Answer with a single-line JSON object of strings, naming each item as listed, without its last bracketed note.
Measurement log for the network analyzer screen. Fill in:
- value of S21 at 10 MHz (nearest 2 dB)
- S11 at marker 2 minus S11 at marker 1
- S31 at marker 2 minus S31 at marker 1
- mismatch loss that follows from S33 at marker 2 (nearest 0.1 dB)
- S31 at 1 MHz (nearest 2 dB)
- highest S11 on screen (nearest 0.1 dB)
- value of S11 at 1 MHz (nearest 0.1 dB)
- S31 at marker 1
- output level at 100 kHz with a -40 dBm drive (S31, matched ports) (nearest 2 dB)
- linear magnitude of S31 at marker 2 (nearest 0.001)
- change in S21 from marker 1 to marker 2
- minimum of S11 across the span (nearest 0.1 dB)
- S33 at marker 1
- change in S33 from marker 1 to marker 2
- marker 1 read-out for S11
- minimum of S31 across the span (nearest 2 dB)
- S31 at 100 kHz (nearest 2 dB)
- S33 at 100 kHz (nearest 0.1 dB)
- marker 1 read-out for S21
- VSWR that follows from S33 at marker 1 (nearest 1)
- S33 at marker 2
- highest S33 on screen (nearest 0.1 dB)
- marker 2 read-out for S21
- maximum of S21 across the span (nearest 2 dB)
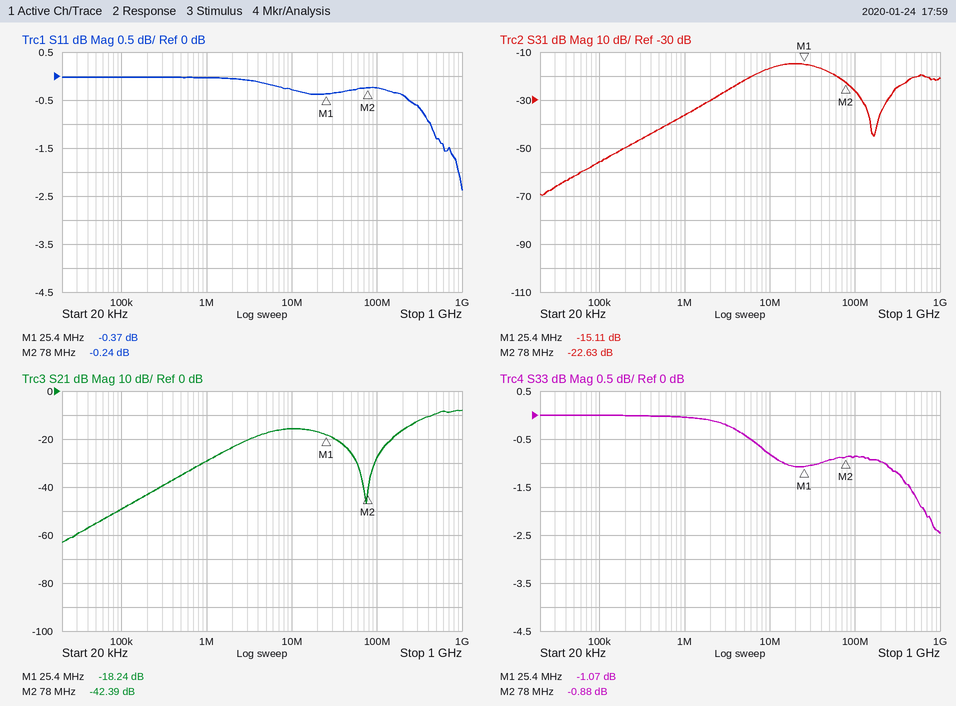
{"value of S21 at 10 MHz": "-16 dB", "S11 at marker 2 minus S11 at marker 1": "0.13 dB", "S31 at marker 2 minus S31 at marker 1": "-7.52 dB", "mismatch loss that follows from S33 at marker 2": "7.4 dB", "S31 at 1 MHz": "-36 dB", "highest S11 on screen": "0.0 dB", "value of S11 at 1 MHz": "0.0 dB", "S31 at marker 1": "-15.11 dB", "output level at 100 kHz with a -40 dBm drive (S31, matched ports)": "-96 dBm", "linear magnitude of S31 at marker 2": "0.074", "change in S21 from marker 1 to marker 2": "-24.15 dB", "minimum of S11 across the span": "-2.4 dB", "S33 at marker 1": "-1.07 dB", "change in S33 from marker 1 to marker 2": "0.19 dB", "marker 1 read-out for S11": "-0.37 dB", "minimum of S31 across the span": "-70 dB", "S31 at 100 kHz": "-56 dB", "S33 at 100 kHz": "0.0 dB", "marker 1 read-out for S21": "-18.24 dB", "VSWR that follows from S33 at marker 1": "16", "S33 at marker 2": "-0.88 dB", "highest S33 on screen": "0.0 dB", "marker 2 read-out for S21": "-42.39 dB", "maximum of S21 across the span": "-8 dB"}
